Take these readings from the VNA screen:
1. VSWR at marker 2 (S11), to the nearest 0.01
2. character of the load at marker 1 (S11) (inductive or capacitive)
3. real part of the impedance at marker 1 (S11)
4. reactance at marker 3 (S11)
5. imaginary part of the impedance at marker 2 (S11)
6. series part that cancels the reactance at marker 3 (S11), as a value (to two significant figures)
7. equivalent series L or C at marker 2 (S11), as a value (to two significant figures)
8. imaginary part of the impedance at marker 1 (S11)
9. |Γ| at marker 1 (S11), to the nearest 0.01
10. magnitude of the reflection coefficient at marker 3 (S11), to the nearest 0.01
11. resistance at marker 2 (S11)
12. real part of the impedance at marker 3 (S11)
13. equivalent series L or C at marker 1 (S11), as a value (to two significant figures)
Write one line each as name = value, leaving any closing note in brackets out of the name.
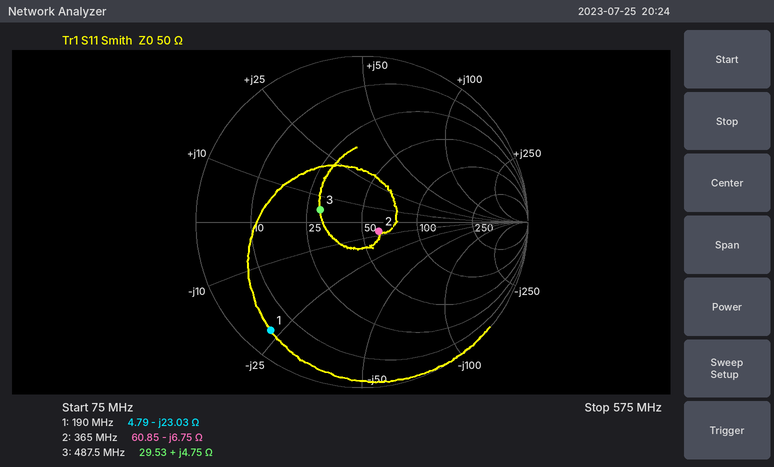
VSWR at marker 2 (S11), to the nearest 0.01 = 1.26
character of the load at marker 1 (S11) = capacitive
real part of the impedance at marker 1 = 4.79 Ω
reactance at marker 3 = +4.75 Ω
imaginary part of the impedance at marker 2 = -6.75 Ω
series part that cancels the reactance at marker 3 (S11), as a value = 69 pF
equivalent series L or C at marker 2 (S11), as a value = 65 pF
imaginary part of the impedance at marker 1 = -23.03 Ω
|Γ| at marker 1 (S11), to the nearest 0.01 = 0.85
magnitude of the reflection coefficient at marker 3 (S11), to the nearest 0.01 = 0.26
resistance at marker 2 = 60.85 Ω
real part of the impedance at marker 3 = 29.53 Ω
equivalent series L or C at marker 1 (S11), as a value = 36 pF
